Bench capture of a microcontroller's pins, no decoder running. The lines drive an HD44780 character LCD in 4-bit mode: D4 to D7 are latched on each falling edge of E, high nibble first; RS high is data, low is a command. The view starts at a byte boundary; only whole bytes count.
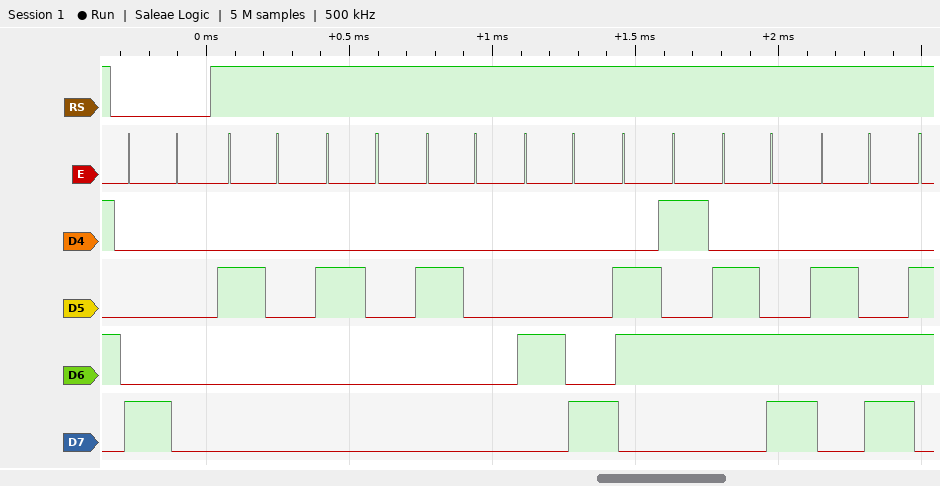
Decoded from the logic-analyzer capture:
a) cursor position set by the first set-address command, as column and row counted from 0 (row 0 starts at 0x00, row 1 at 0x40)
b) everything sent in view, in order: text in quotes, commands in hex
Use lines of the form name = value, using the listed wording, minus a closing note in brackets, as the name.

cursor position set by the first set-address command, as column and row counted from 0 = column 0, row 0
everything sent in view, in order: text in quotes, commands in hex = 0x80 "   Hell"
